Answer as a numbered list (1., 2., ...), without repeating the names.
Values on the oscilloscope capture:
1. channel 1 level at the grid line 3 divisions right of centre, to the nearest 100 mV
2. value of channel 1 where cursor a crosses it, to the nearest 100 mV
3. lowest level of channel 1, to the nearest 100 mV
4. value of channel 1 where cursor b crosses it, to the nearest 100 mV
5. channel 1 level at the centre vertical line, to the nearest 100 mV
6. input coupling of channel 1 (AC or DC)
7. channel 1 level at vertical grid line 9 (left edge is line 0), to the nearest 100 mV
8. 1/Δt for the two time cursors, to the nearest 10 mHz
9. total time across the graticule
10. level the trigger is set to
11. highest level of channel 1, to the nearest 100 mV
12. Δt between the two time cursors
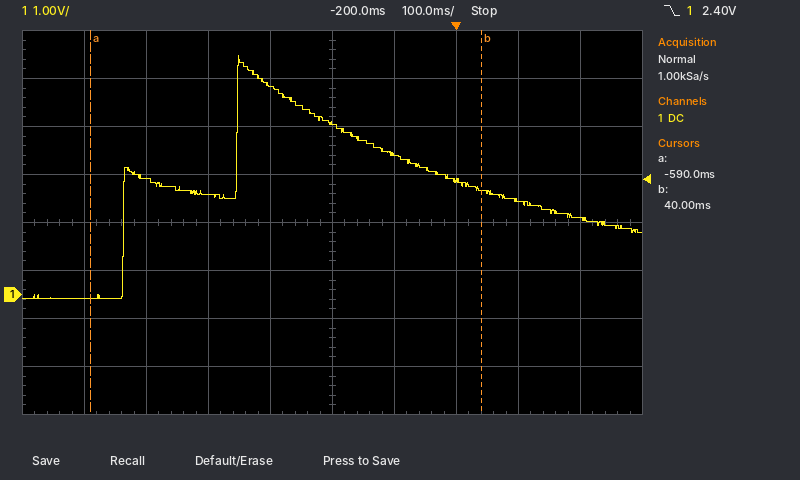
1. 2.0 V
2. -100 mV
3. -100 mV
4. 2.2 V
5. 3.6 V
6. DC
7. 1.6 V
8. 1.59 Hz
9. 1 s
10. 2.40 V
11. 5.0 V
12. 630 ms
